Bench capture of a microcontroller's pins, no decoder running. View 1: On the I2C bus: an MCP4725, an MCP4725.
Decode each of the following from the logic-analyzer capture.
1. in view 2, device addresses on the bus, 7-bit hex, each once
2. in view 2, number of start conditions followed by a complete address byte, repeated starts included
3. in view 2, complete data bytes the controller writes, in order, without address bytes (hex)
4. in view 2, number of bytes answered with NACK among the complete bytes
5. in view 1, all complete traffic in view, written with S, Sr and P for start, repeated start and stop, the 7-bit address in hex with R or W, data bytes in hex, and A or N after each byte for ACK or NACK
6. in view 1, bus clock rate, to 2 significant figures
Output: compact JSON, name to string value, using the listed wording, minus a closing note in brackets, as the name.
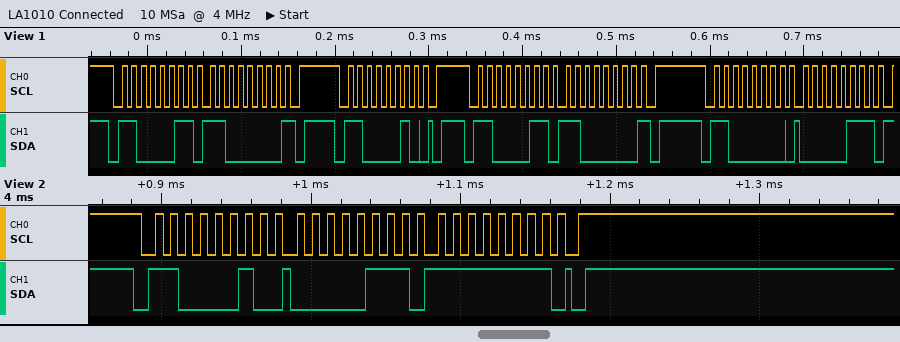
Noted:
{"in view 2, device addresses on the bus, 7-bit hex, each once": "0x61", "in view 2, number of start conditions followed by a complete address byte, repeated starts included": "1", "in view 2, complete data bytes the controller writes, in order, without address bytes": "07 FF", "in view 2, number of bytes answered with NACK among the complete bytes": "0", "in view 1, all complete traffic in view, written with S, Sr and P for start, repeated start and stop, the 7-bit address in hex with R or W, data bytes in hex, and A or N after each byte for ACK or NACK": "S 61R A C0 N P S 61W A P S 61R A C0 N P S 60W A 07 A", "in view 1, bus clock rate, to 2 significant figures": "100 kHz"}
